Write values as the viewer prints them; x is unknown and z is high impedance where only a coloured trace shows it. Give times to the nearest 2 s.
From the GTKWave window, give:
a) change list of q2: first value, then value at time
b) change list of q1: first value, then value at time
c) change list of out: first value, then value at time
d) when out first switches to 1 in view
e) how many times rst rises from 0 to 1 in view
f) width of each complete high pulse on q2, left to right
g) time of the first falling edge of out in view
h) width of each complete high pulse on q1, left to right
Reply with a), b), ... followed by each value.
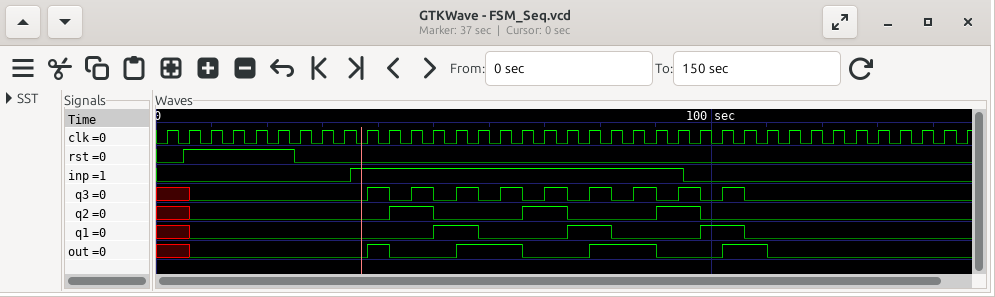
a) x, 0 at 6 s, 1 at 42 s, 0 at 50 s, 1 at 66 s, 0 at 74 s, 1 at 90 s, 0 at 98 s
b) x, 0 at 6 s, 1 at 50 s, 0 at 58 s, 1 at 74 s, 0 at 82 s, 1 at 98 s, 0 at 106 s
c) x, 0 at 6 s, 1 at 38 s, 0 at 42 s, 1 at 54 s, 0 at 66 s, 1 at 78 s, 0 at 90 s, 1 at 102 s, 0 at 110 s
d) 38 s
e) 1
f) 8 s, 8 s, 8 s
g) 42 s
h) 8 s, 8 s, 8 s
